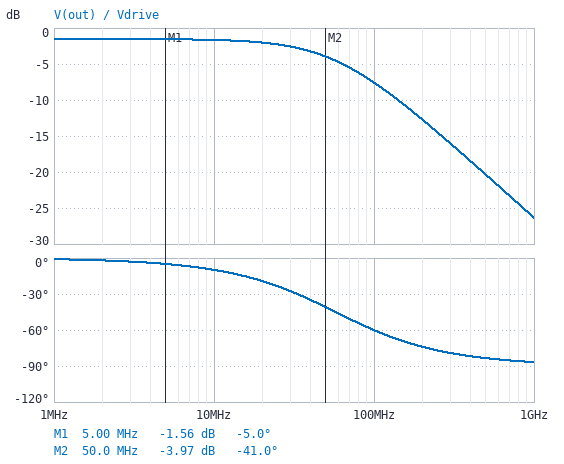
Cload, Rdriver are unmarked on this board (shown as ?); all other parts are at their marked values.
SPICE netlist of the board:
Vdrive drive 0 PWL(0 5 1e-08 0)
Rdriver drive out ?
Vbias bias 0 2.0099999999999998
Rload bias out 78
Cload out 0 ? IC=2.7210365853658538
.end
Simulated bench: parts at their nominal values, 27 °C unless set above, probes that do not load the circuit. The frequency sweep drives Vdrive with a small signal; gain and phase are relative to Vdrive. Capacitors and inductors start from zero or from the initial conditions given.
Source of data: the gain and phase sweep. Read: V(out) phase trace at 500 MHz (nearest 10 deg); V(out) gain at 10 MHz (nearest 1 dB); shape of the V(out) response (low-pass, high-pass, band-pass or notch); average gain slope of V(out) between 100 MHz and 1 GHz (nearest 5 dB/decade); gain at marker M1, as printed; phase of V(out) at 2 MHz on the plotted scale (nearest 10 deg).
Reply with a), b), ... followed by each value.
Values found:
a) -80 deg
b) -2 dB
c) low-pass
d) -20 dB/decade
e) -1.56 dB
f) 0 deg
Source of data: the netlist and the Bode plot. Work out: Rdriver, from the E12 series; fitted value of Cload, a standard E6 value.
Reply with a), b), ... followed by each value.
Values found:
a) 15 Ω
b) 220 pF
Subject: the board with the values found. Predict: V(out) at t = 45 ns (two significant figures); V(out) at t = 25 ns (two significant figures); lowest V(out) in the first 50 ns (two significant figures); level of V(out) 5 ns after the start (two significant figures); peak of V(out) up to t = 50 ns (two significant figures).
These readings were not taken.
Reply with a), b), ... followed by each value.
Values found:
a) 320 mV
b) 330 mV
c) 320 mV
d) 3.1 V
e) 3.4 V
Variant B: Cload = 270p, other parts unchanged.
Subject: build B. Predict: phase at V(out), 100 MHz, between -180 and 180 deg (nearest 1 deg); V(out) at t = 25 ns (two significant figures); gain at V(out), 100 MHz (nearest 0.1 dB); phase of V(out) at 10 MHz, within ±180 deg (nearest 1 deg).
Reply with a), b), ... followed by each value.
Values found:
a) -65 deg
b) 340 mV
c) -9.0 dB
d) -12 deg
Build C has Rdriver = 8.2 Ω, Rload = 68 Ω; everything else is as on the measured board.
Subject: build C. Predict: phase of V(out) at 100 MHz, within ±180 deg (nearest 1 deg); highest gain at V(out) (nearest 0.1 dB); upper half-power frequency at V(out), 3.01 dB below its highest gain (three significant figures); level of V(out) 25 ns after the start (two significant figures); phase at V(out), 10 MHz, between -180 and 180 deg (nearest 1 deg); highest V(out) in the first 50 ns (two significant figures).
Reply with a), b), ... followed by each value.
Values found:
a) -45 deg
b) -1.0 dB
c) 98.9 MHz
d) 220 mV
e) -6 deg
f) 3.7 V
